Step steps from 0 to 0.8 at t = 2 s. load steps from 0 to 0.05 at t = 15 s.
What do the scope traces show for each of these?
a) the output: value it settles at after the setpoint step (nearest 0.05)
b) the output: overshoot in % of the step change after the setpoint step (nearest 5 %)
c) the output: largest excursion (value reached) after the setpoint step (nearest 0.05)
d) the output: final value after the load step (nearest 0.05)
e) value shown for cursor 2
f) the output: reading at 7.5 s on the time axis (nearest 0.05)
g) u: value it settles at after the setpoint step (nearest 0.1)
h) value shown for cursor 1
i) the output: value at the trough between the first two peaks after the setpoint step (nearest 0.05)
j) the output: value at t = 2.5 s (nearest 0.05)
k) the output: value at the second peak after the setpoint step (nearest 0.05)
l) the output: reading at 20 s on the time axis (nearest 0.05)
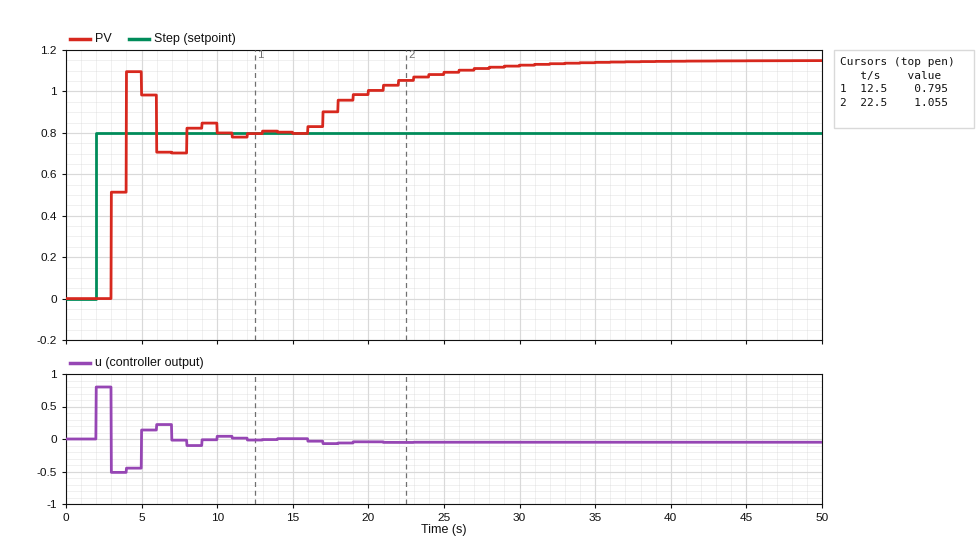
0.80
35 %
1.10
1.15
1.055
0.70
0.0
0.795
0.70
0.00
0.85
1.00
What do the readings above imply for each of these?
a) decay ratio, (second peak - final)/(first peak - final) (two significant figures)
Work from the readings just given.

0.17
